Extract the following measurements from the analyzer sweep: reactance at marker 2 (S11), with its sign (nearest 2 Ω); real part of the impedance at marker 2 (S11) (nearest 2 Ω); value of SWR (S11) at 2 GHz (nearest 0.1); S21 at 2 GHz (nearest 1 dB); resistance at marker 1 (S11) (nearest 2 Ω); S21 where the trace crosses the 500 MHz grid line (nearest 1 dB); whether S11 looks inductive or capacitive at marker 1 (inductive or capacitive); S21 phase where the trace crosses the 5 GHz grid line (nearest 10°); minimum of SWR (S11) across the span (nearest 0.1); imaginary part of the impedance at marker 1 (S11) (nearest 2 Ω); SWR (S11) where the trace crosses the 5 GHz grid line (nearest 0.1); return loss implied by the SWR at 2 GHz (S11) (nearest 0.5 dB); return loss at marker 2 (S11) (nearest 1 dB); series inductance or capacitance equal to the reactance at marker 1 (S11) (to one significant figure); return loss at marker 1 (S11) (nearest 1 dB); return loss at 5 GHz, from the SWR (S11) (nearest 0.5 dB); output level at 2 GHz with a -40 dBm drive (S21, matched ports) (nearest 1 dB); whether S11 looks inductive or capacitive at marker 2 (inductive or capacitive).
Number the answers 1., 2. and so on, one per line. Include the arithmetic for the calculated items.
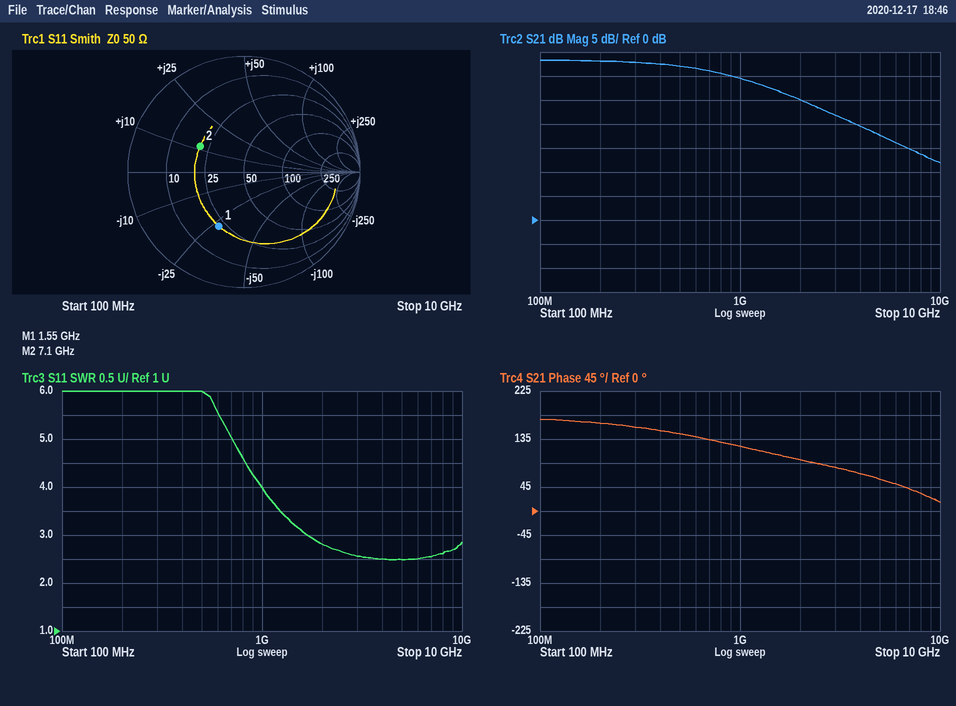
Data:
1. +12 Ω
2. 20 Ω
3. 2.8
4. 25 dB
5. 22 Ω
6. 32 dB
7. capacitive
8. 60°
9. 2.5
10. -28 Ω
11. 2.5
12. −20 log10((2.8 − 1)/(2.8 + 1)) ≈ 6.5 dB
13. 7 dB
14. C = 1/(2π × 1.55 GHz × 28 Ω) ≈ 4 pF
15. 6 dB
16. −20 log10((2.5 − 1)/(2.5 + 1)) ≈ 7.36 dB, so 7.5 dB to the nearest 0.5 dB
17. -40 dBm + (25 dB) = -15 dBm
18. inductive
